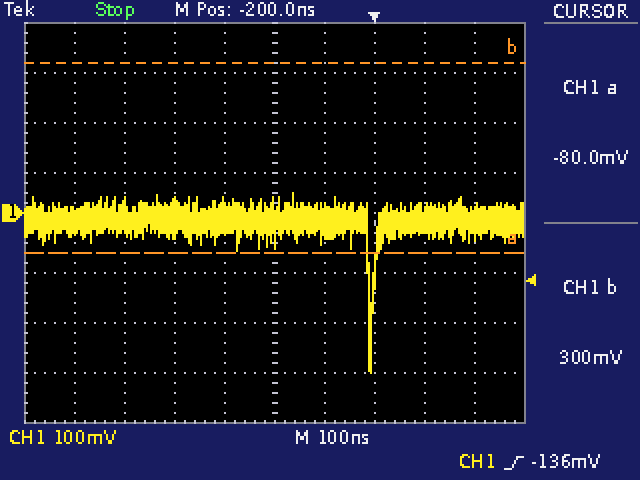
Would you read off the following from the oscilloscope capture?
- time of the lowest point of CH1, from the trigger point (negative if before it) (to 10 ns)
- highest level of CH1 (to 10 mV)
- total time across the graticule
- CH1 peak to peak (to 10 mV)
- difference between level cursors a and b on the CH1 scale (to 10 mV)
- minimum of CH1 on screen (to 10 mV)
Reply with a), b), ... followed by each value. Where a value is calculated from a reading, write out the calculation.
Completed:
a) -10 ns
b) 40 mV
c) 1 µs
d) 40 mV − (-320 mV) = 360 mV
e) 380 mV
f) -320 mV
